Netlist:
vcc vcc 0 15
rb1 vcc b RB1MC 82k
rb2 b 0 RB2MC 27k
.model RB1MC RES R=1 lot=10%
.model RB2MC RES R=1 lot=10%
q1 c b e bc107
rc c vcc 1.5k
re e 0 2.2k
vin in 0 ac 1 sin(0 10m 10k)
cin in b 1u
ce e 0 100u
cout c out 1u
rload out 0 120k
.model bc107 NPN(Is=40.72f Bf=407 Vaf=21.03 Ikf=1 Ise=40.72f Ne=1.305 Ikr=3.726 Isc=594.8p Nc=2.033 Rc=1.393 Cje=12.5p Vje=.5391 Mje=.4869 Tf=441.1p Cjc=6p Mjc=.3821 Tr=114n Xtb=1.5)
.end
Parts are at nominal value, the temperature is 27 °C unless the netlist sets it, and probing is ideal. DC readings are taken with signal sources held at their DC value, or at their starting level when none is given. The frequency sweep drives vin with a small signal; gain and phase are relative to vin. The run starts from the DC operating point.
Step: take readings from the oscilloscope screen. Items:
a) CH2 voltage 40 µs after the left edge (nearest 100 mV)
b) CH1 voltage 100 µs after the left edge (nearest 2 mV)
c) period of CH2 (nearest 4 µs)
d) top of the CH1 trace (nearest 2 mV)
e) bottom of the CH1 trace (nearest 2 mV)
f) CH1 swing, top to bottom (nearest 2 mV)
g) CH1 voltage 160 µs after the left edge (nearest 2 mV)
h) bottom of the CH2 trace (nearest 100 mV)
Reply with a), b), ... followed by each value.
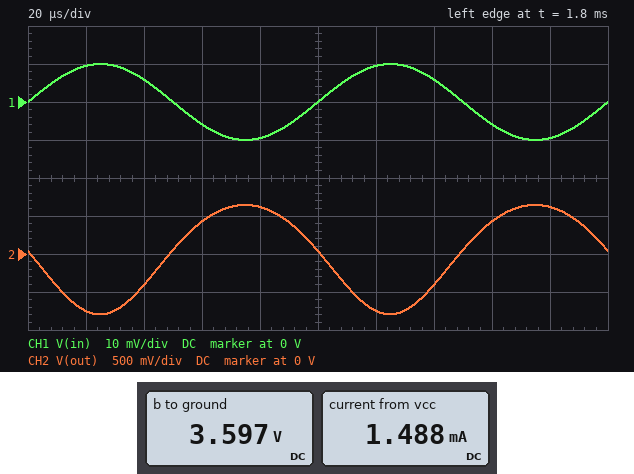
a) -400 mV
b) 0 V
c) 100 µs
d) 10 mV
e) -10 mV
f) 20 mV
g) -6 mV
h) -800 mV
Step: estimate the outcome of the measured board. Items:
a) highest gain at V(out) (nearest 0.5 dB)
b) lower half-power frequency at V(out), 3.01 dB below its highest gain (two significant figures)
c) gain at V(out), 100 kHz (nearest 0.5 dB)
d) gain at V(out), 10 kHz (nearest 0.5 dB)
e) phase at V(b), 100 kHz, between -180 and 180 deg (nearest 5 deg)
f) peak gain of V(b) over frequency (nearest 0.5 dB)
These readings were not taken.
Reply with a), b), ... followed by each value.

a) 37.0 dB
b) 110 Hz
c) 37.0 dB
d) 37.0 dB
e) 0 deg
f) 0 dB
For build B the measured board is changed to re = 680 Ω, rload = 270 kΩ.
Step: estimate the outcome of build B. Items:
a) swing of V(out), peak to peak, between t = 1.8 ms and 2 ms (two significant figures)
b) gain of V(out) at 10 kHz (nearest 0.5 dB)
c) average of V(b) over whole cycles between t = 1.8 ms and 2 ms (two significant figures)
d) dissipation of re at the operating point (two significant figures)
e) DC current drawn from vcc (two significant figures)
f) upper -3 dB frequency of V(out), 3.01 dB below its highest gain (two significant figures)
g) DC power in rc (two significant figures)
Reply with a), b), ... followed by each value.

a) 3.7 V
b) 45.5 dB
c) 3.4 V
d) 11 mW
e) 4.1 mA
f) 49 MHz
g) 24 mW
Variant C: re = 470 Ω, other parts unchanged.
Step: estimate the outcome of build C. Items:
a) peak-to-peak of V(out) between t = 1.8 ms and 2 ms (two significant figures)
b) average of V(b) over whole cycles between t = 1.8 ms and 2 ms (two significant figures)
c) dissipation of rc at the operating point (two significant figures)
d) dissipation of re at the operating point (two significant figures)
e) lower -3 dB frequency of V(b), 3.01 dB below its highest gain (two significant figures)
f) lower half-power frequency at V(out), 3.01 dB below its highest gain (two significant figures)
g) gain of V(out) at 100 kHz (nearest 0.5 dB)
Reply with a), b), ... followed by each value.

a) 4.6 V
b) 3.2 V
c) 45 mW
d) 14 mW
e) 130 Hz
f) 390 Hz
g) 47.5 dB
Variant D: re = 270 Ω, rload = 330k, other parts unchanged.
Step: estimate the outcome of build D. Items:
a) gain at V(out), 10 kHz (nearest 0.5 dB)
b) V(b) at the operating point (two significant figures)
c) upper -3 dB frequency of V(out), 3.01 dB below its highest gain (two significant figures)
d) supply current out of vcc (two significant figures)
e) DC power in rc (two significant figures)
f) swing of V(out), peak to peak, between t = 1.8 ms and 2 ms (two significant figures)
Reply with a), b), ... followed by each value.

a) 49.5 dB
b) 2.9 V
c) 24 MHz
d) 8.4 mA
e) 100 mW
f) 4.9 V
